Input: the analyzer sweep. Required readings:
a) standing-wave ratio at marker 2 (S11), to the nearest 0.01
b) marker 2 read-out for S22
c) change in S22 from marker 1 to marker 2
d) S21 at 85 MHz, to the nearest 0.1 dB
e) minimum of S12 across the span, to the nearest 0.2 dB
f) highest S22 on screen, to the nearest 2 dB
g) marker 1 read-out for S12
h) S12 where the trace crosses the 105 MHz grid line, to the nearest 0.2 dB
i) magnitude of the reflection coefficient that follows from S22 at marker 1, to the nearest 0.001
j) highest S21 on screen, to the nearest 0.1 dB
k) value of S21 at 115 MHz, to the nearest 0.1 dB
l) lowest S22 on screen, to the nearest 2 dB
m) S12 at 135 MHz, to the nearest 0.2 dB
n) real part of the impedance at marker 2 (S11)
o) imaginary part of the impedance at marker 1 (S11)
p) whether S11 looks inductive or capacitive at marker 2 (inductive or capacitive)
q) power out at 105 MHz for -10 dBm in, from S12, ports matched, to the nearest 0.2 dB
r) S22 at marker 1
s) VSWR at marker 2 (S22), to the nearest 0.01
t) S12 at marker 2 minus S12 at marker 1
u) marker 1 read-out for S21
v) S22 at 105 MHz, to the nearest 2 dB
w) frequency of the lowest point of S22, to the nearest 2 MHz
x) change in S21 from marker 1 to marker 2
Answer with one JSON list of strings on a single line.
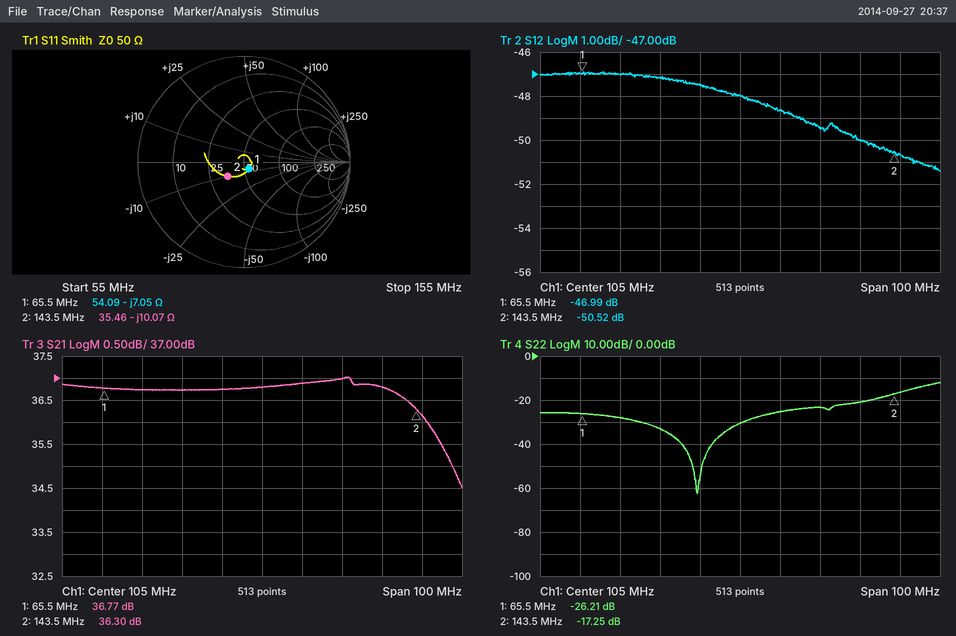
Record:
["1.52", "-17.25 dB", "8.96 dB", "36.7 dB", "-51.4 dB", "-12 dB", "-46.99 dB", "-48.0 dB", "0.049", "37.0 dB", "36.9 dB", "-62 dB", "-50.0 dB", "35.46 Ω", "-7.05 Ω", "capacitive", "-58.0 dBm", "-26.21 dB", "1.32", "-3.53 dB", "36.77 dB", "-30 dB", "94 MHz", "-0.47 dB"]
